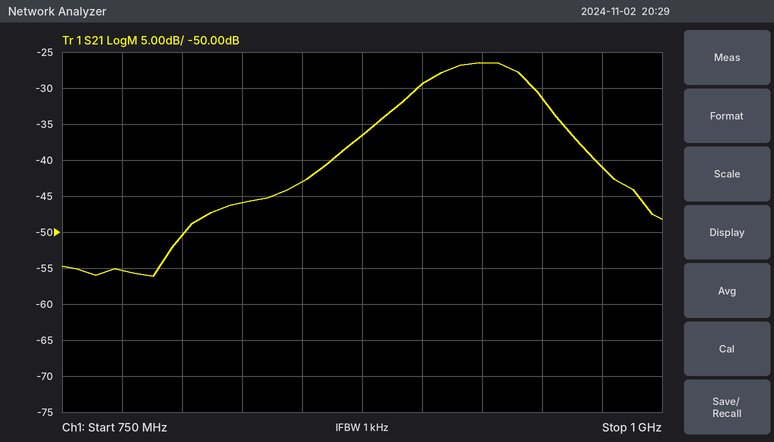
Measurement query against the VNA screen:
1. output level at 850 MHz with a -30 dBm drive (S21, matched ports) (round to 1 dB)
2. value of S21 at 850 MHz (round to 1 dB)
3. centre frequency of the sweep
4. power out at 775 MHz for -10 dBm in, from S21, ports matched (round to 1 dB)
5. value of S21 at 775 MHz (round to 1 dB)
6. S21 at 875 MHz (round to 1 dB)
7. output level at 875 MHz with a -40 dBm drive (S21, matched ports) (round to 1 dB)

-73 dBm
-43 dB
875 MHz
-65 dBm
-55 dB
-37 dB
-77 dBm
